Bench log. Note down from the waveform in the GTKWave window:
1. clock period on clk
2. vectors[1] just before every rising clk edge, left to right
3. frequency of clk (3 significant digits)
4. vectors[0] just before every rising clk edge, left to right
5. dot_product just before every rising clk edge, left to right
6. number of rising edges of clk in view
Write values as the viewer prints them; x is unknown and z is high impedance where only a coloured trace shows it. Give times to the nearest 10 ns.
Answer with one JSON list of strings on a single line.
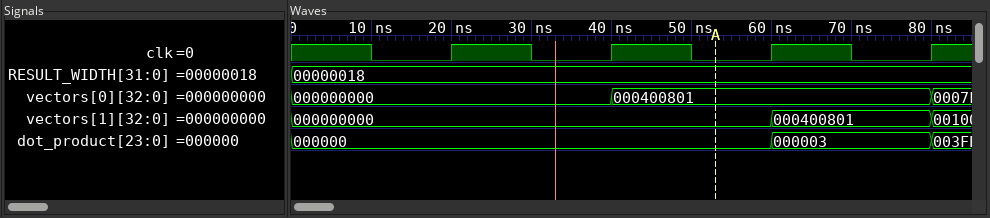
["20 ns", "000000000, 000000000, 000000000, 000400801", "50.0 MHz", "000000000, 000000000, 000400801, 000400801", "000000, 000000, 000000, 000003", "4"]
